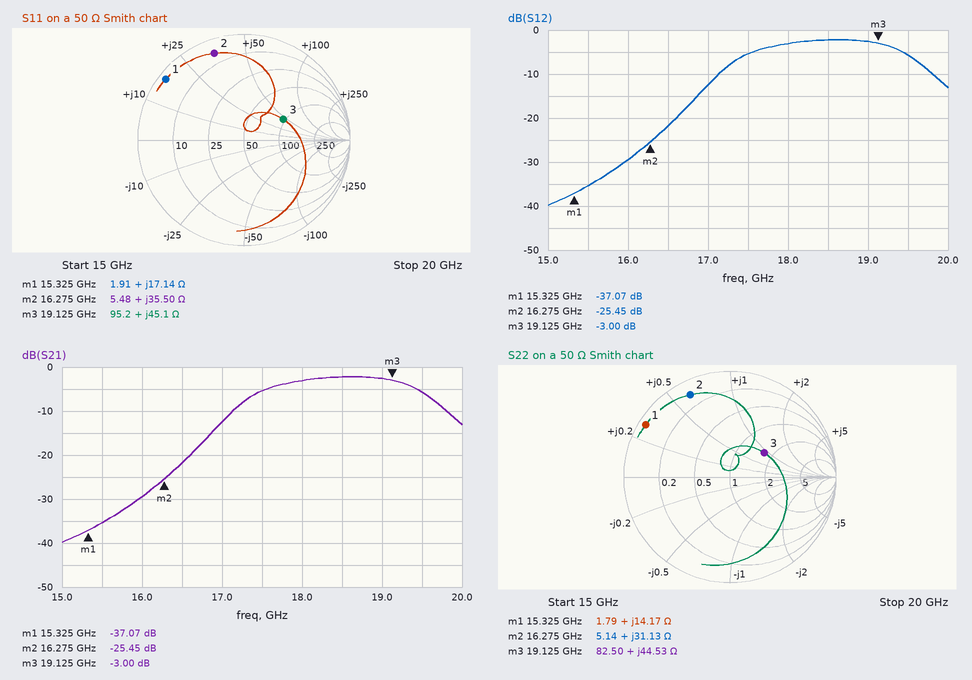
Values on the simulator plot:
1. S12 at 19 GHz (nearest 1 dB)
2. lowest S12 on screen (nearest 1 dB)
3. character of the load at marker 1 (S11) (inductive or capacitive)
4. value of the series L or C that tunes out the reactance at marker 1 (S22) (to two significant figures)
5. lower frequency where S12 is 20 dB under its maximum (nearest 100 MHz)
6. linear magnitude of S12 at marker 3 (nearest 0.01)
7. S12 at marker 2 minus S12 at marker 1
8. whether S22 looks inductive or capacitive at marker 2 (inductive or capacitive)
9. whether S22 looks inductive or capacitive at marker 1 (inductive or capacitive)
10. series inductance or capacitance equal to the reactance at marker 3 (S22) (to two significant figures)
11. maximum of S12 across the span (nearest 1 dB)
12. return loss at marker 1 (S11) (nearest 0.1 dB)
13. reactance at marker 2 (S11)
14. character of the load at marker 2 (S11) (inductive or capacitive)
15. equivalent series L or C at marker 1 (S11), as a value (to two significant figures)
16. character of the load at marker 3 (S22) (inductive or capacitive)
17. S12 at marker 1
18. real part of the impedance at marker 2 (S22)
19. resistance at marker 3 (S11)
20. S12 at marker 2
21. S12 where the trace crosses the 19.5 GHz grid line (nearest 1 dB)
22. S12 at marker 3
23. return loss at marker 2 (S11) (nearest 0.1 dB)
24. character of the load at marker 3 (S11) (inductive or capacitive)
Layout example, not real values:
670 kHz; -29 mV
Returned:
-3 dB; -40 dB; inductive; 730 fF; 16.5 GHz; 0.71; 11.62 dB; inductive; inductive; 370 pH; -2 dB; 0.6 dB; +35.50 Ω; inductive; 180 pH; inductive; -37.07 dB; 5.14 Ω; 95.2 Ω; -25.45 dB; -6 dB; -3.00 dB; 1.3 dB; inductive
